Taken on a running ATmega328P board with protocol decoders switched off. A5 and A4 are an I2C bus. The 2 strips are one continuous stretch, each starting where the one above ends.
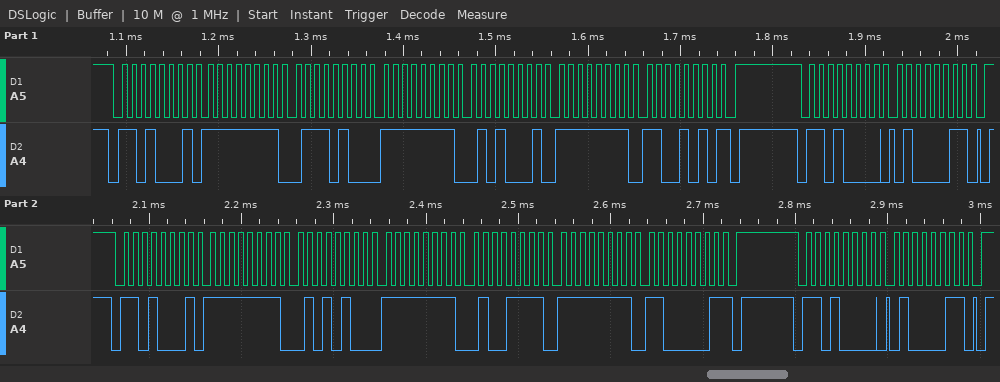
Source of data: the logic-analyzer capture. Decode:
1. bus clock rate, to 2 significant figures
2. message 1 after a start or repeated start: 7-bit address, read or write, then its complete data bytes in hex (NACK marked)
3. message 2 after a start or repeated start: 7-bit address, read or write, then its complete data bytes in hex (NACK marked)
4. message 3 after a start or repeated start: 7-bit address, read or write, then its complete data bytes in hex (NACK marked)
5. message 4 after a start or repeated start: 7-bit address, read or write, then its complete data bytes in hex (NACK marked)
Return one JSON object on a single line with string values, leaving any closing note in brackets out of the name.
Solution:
{"bus clock rate, to 2 significant figures": "100 kHz", "message 1 after a start or repeated start: 7-bit address, read or write, then its complete data bytes in hex": "0x68 read: FF 74 FF 51 FF CA NACK", "message 2 after a start or repeated start: 7-bit address, read or write, then its complete data bytes in hex": "0x68 write: 43", "message 3 after a start or repeated start: 7-bit address, read or write, then its complete data bytes in hex": "0x68 read: FF 54 FF 4F FF C1 NACK", "message 4 after a start or repeated start: 7-bit address, read or write, then its complete data bytes in hex": "0x68 write: 43"}
